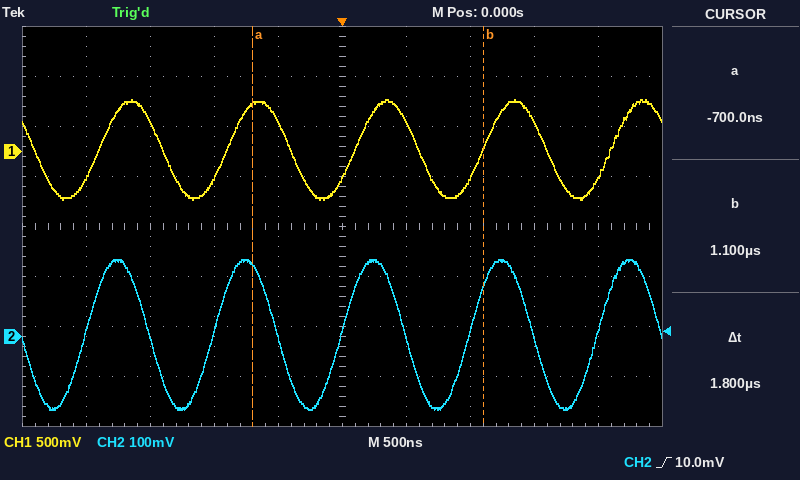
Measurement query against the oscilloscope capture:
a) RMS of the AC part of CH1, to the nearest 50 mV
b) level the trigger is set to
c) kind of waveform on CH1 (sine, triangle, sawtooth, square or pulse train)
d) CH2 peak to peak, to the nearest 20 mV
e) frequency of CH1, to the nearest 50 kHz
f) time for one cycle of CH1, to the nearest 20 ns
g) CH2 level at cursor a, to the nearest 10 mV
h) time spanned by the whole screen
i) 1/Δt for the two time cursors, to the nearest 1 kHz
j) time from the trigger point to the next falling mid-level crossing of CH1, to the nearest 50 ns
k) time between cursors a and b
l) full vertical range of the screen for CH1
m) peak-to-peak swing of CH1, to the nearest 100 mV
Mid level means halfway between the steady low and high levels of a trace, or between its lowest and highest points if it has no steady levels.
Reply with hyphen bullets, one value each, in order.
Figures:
- 350 mV
- 10.0 mV
- sine
- 300 mV
- 1.00 MHz
- 1.00 µs
- 140 mV
- 5 µs
- 556 kHz
- 600 ns
- 1.8 µs
- 4 V
- 1.00 V
